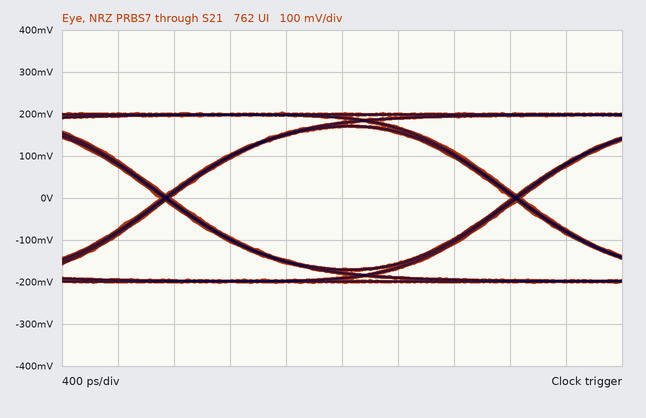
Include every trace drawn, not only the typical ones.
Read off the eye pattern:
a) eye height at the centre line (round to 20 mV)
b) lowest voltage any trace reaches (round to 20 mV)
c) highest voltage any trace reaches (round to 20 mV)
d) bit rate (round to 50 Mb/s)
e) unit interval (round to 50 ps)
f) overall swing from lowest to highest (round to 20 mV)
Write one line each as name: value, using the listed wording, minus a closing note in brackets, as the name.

eye height at the centre line: 340 mV
lowest voltage any trace reaches: -200 mV
highest voltage any trace reaches: 200 mV
bit rate: 400 Mb/s
unit interval: 2.50 ns
overall swing from lowest to highest: 400 mV
